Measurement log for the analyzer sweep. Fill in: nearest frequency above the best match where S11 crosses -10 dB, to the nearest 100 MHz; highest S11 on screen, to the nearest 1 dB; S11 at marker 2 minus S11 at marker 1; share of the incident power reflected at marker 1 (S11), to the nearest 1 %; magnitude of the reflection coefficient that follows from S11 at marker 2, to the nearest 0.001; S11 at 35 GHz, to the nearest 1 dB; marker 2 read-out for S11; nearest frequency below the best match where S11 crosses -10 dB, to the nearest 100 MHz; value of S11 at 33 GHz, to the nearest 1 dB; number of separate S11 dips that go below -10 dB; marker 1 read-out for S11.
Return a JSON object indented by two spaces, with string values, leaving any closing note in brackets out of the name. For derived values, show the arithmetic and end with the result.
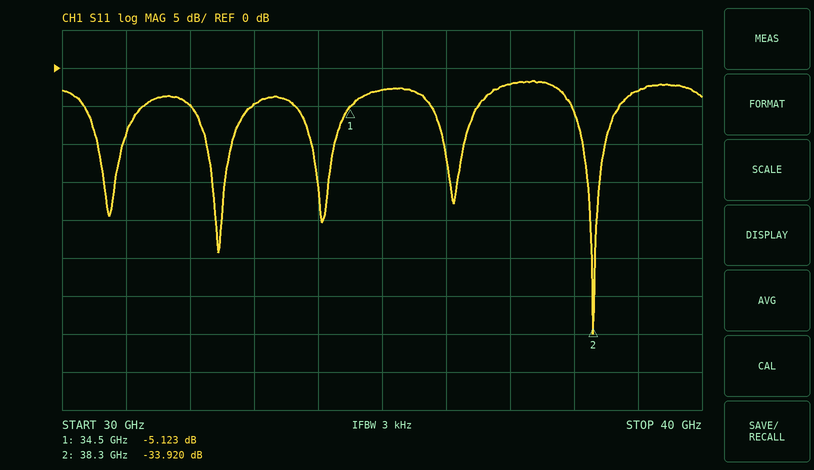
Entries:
{
  "nearest frequency above the best match where S11 crosses -10 dB, to the nearest 100 MHz": "38.5 GHz",
  "highest S11 on screen, to the nearest 1 dB": "-2 dB",
  "S11 at marker 2 minus S11 at marker 1": "-33.92 − (-5.123) = -28.797 dB",
  "share of the incident power reflected at marker 1 (S11), to the nearest 1 %": "10^(-5.123/10) ≈ 31 %",
  "magnitude of the reflection coefficient that follows from S11 at marker 2, to the nearest 0.001": "10^(-33.92/20) ≈ 0.020",
  "S11 at 35 GHz, to the nearest 1 dB": "-3 dB",
  "marker 2 read-out for S11": "-33.920 dB",
  "nearest frequency below the best match where S11 crosses -10 dB, to the nearest 100 MHz": "38.1 GHz",
  "value of S11 at 33 GHz, to the nearest 1 dB": "-5 dB",
  "number of separate S11 dips that go below -10 dB": "5",
  "marker 1 read-out for S11": "-5.123 dB"
}
